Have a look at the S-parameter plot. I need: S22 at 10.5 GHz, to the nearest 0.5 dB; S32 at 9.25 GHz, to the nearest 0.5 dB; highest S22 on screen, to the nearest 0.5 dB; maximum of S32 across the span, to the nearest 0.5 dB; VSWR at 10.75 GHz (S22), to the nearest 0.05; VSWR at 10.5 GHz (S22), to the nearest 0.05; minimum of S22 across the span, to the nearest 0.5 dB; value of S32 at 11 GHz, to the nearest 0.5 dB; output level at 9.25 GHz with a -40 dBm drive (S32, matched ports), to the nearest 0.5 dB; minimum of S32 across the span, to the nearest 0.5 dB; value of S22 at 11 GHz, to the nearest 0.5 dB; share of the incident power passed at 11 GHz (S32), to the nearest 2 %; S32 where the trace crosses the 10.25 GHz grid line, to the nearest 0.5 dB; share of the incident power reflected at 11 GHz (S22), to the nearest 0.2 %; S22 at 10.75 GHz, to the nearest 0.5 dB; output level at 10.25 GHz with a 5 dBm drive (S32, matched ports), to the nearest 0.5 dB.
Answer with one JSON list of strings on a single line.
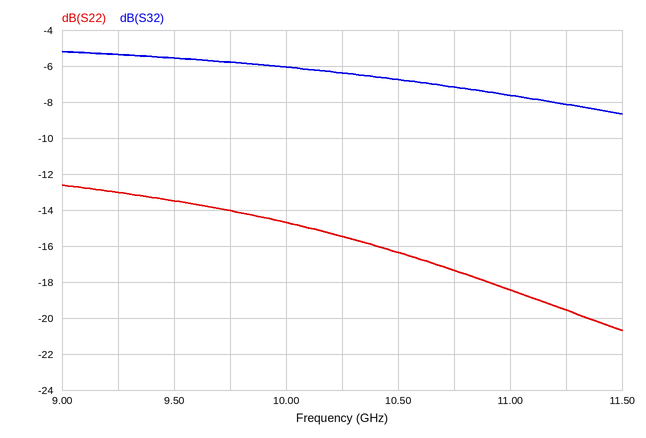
["-16.5 dB", "-5.5 dB", "-12.5 dB", "-5.0 dB", "1.30", "1.35", "-20.5 dB", "-7.5 dB", "-45.5 dBm", "-8.5 dB", "-18.5 dB", "18 %", "-6.5 dB", "1.4 %", "-17.5 dB", "-1.5 dBm"]
